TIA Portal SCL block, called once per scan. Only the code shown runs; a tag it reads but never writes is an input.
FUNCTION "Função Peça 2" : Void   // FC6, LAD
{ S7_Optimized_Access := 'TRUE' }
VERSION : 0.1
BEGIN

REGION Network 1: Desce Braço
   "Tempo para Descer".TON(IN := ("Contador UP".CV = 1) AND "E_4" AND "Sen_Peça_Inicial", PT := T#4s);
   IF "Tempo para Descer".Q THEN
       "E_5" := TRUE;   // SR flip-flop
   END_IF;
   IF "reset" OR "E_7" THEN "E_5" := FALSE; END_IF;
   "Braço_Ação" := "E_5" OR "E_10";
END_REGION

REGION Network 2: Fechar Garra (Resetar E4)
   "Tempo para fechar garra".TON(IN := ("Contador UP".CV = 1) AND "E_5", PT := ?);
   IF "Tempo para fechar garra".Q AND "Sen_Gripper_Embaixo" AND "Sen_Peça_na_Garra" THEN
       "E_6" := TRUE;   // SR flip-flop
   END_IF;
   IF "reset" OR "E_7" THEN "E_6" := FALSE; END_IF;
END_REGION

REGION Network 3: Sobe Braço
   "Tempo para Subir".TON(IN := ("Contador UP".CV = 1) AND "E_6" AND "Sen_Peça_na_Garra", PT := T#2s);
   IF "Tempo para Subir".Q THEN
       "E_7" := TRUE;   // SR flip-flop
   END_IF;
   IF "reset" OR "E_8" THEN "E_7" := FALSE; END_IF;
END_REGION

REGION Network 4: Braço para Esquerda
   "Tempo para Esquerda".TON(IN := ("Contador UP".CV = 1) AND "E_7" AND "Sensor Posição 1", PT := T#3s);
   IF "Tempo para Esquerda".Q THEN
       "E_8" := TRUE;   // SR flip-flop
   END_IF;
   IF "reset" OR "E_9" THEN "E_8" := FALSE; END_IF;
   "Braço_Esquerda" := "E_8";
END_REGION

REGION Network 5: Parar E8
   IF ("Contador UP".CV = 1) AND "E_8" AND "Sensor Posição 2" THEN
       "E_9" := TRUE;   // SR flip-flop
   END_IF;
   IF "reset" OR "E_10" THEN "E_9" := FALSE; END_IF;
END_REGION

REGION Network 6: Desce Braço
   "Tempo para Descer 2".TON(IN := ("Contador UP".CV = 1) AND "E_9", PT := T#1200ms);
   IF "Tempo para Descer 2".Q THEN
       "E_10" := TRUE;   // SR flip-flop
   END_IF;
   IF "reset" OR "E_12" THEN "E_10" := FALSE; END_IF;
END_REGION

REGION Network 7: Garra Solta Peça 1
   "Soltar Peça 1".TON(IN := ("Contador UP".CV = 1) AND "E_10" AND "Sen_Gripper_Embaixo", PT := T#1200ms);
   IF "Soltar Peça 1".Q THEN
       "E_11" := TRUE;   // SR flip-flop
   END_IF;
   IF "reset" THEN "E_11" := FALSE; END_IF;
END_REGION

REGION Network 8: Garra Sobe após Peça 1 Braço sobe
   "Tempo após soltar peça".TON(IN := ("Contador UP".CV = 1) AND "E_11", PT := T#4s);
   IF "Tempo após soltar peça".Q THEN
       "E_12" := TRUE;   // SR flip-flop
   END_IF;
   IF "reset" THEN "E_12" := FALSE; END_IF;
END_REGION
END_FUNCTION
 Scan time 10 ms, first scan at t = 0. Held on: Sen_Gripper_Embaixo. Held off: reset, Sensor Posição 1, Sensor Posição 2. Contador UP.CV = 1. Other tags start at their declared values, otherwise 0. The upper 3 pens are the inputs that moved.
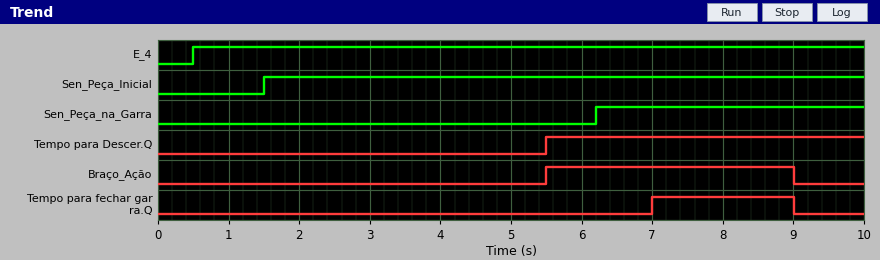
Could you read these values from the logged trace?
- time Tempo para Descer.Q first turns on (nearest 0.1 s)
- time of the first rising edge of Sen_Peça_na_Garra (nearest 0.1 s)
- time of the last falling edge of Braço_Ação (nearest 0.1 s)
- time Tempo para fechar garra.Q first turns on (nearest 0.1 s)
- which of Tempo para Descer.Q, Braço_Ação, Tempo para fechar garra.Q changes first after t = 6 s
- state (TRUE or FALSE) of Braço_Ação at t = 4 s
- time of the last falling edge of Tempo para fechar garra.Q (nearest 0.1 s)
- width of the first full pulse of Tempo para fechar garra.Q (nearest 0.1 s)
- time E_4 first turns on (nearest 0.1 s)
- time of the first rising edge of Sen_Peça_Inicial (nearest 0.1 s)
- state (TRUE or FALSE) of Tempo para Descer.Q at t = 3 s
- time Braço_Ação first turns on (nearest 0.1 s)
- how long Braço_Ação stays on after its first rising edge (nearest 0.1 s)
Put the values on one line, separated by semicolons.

5.5 s; 6.2 s; 9.0 s; 7.0 s; Tempo para fechar garra.Q; FALSE; 9.0 s; 2.0 s; 0.5 s; 1.5 s; FALSE; 5.5 s; 3.5 s
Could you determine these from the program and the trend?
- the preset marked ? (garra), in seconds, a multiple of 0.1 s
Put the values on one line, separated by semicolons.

1.5 s
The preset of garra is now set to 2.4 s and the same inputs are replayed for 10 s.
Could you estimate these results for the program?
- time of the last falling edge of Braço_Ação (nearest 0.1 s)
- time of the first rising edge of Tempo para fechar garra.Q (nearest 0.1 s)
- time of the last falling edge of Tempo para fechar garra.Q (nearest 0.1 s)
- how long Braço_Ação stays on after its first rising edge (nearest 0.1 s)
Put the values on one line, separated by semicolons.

9.9 s; 7.9 s; 9.9 s; 4.4 s
